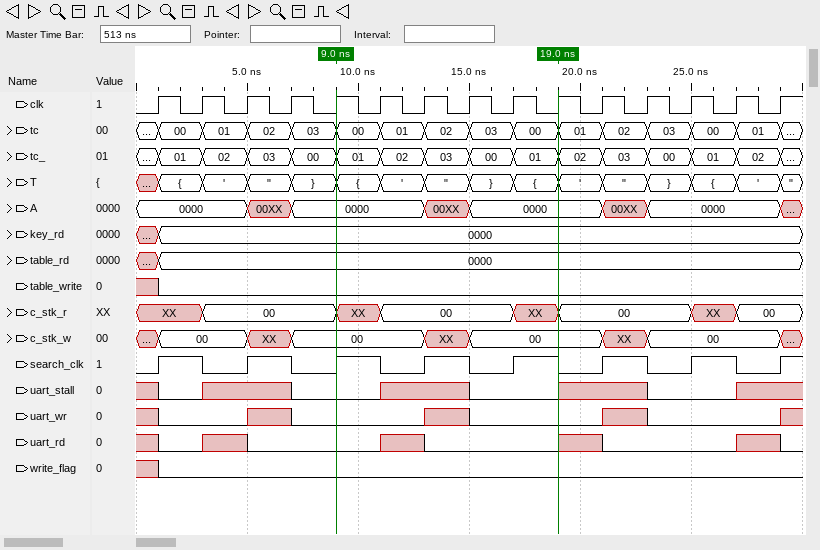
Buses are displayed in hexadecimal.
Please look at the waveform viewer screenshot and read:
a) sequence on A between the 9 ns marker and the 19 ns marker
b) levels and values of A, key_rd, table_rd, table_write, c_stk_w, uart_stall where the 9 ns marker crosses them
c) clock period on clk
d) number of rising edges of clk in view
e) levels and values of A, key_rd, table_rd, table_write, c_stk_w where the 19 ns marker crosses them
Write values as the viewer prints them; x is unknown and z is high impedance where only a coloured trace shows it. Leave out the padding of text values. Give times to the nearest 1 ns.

0000, 00XX, 0000
A=0000, key_rd=0000, table_rd=0000, table_write=0, c_stk_w=00, uart_stall=0
2 ns
15
A=0000, key_rd=0000, table_rd=0000, table_write=0, c_stk_w=00
